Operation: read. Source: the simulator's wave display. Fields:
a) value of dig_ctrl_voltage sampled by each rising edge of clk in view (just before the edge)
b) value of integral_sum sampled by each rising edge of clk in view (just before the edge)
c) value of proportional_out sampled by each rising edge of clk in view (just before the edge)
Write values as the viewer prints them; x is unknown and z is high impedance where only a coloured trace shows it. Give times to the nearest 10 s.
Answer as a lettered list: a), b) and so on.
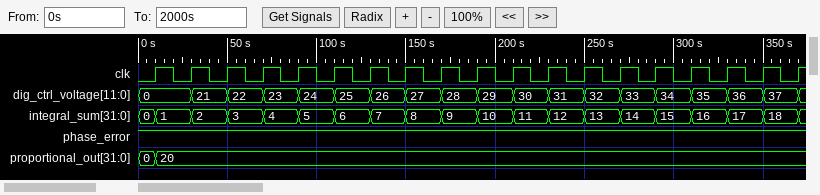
a) 0, 0, 21, 22, 23, 24, 25, 26, 27, 28, 29, 30, 31, 32, 33, 34, 35, 36, 37
b) 0, 1, 2, 3, 4, 5, 6, 7, 8, 9, 10, 11, 12, 13, 14, 15, 16, 17, 18
c) 0, 20, 20, 20, 20, 20, 20, 20, 20, 20, 20, 20, 20, 20, 20, 20, 20, 20, 20
